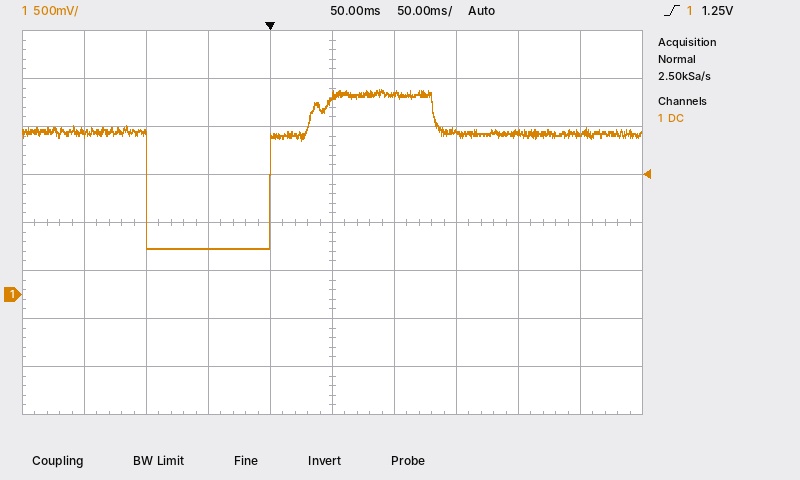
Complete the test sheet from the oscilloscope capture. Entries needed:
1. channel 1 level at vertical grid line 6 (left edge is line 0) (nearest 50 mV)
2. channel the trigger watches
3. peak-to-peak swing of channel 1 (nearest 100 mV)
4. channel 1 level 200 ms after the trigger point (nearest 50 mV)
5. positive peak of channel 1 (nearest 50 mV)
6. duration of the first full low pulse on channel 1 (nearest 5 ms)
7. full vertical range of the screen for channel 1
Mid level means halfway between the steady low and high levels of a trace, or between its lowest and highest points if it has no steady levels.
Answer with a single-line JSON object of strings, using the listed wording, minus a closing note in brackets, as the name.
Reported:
{"channel 1 level at vertical grid line 6 (left edge is line 0)": "2.10 V", "channel the trigger watches": "channel 1", "peak-to-peak swing of channel 1": "1.70 V", "channel 1 level 200 ms after the trigger point": "1.70 V", "positive peak of channel 1": "2.15 V", "duration of the first full low pulse on channel 1": "100 ms", "full vertical range of the screen for channel 1": "4 V"}
